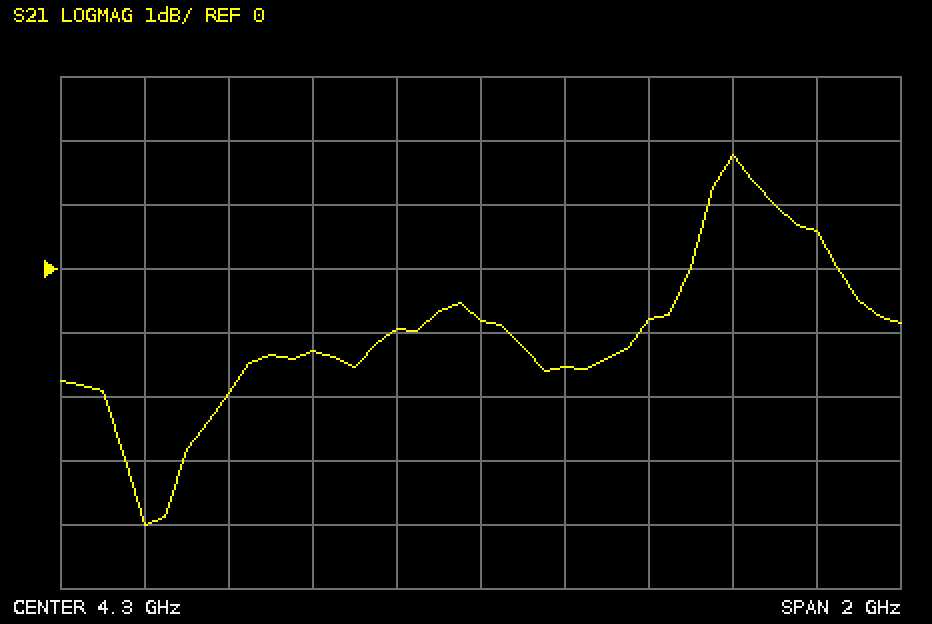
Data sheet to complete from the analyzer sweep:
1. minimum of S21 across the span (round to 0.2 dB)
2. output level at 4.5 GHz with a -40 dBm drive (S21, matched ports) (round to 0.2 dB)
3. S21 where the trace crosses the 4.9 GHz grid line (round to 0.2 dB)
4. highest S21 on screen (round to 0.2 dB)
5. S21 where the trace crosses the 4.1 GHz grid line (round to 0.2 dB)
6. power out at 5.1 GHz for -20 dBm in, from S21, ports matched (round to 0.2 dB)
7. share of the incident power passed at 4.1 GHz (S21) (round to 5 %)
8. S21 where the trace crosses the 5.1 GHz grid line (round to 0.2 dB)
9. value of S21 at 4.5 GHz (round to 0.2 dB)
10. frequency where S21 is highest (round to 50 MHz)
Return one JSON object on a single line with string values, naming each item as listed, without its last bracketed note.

{"minimum of S21 across the span": "-4.0 dB", "output level at 4.5 GHz with a -40 dBm drive (S21, matched ports)": "-41.6 dBm", "S21 where the trace crosses the 4.9 GHz grid line": "1.8 dB", "highest S21 on screen": "1.8 dB", "S21 where the trace crosses the 4.1 GHz grid line": "-1.0 dB", "power out at 5.1 GHz for -20 dBm in, from S21, ports matched": "-19.4 dBm", "share of the incident power passed at 4.1 GHz (S21)": "80 %", "S21 where the trace crosses the 5.1 GHz grid line": "0.6 dB", "value of S21 at 4.5 GHz": "-1.6 dB", "frequency where S21 is highest": "4.90 GHz"}
